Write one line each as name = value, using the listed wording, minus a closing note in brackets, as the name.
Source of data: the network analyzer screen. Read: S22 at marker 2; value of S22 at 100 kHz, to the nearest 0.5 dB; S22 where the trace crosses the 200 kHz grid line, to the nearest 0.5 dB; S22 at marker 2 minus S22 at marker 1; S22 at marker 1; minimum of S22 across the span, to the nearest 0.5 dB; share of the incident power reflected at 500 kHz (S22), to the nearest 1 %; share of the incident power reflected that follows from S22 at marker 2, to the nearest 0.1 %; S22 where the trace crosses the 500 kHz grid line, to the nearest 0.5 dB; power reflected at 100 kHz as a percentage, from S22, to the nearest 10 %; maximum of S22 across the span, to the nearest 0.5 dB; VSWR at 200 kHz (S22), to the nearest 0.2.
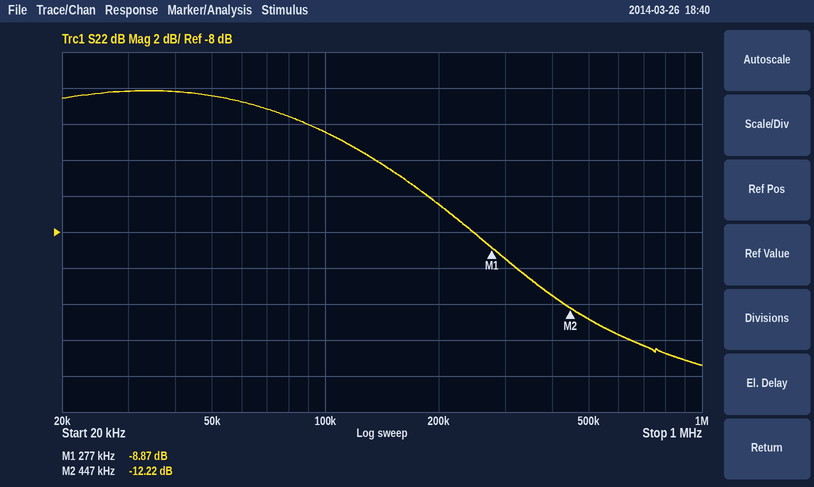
S22 at marker 2 = -12.22 dB
value of S22 at 100 kHz, to the nearest 0.5 dB = -2.5 dB
S22 where the trace crosses the 200 kHz grid line, to the nearest 0.5 dB = -6.5 dB
S22 at marker 2 minus S22 at marker 1 = -3.35 dB
S22 at marker 1 = -8.87 dB
minimum of S22 across the span, to the nearest 0.5 dB = -15.5 dB
share of the incident power reflected at 500 kHz (S22), to the nearest 1 % = 5 %
share of the incident power reflected that follows from S22 at marker 2, to the nearest 0.1 % = 6.0 %
S22 where the trace crosses the 500 kHz grid line, to the nearest 0.5 dB = -13.0 dB
power reflected at 100 kHz as a percentage, from S22, to the nearest 10 % = 60 %
maximum of S22 across the span, to the nearest 0.5 dB = 0.0 dB
VSWR at 200 kHz (S22), to the nearest 0.2 = 2.8
